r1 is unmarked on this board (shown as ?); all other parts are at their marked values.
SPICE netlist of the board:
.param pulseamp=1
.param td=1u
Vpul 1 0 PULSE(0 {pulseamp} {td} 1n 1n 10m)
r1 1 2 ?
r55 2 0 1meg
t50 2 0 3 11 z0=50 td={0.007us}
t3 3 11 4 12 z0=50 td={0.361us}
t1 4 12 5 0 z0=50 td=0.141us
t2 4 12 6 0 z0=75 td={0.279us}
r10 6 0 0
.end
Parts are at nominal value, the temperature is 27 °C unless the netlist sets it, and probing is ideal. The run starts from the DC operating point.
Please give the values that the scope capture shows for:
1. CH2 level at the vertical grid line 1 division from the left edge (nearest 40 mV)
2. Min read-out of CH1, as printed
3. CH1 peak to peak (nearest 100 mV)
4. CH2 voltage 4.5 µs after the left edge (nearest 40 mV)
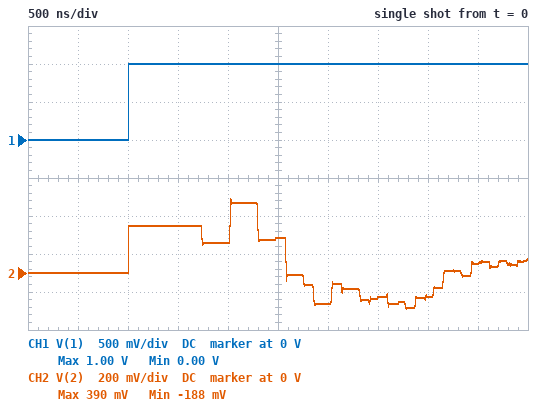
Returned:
0 V
0.00 V
1.0 V
40 mV
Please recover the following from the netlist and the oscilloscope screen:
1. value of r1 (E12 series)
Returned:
150 Ω
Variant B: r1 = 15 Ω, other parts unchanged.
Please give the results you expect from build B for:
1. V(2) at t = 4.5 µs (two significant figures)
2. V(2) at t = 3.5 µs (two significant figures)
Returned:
230 mV
400 mV
